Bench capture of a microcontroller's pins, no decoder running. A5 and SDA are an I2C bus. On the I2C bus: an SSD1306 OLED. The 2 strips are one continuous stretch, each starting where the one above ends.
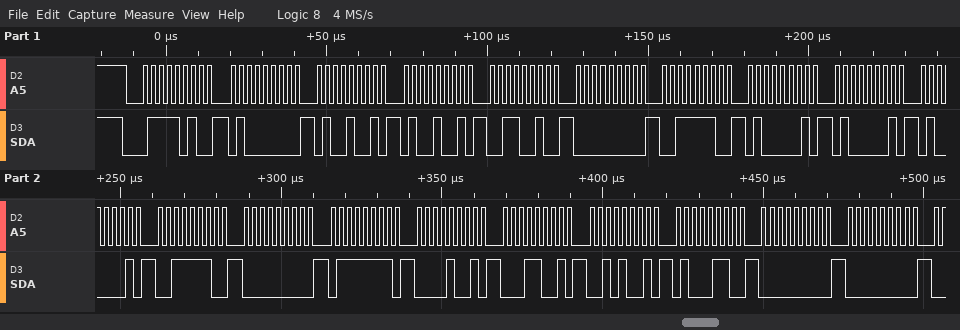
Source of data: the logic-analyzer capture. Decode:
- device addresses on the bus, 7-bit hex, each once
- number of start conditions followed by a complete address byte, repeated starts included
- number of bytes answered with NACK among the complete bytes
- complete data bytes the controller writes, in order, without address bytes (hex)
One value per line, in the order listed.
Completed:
0x3D
1
0
40 49 49 32 00 3E 41 41 41 3E 00 7F 09 19 29 46 00 00
